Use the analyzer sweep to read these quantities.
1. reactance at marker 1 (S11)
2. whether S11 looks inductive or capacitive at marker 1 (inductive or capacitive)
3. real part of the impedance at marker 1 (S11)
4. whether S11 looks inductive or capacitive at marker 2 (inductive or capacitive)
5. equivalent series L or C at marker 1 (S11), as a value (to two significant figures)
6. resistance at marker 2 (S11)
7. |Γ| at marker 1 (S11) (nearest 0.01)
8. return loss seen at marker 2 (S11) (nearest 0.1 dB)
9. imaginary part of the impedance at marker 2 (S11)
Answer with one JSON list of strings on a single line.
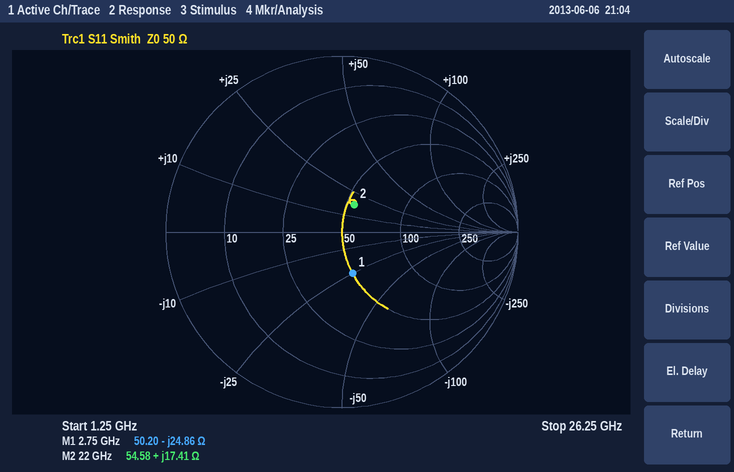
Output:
["-24.86 Ω", "capacitive", "50.20 Ω", "inductive", "2.3 pF", "54.58 Ω", "0.24", "15.4 dB", "+17.41 Ω"]
